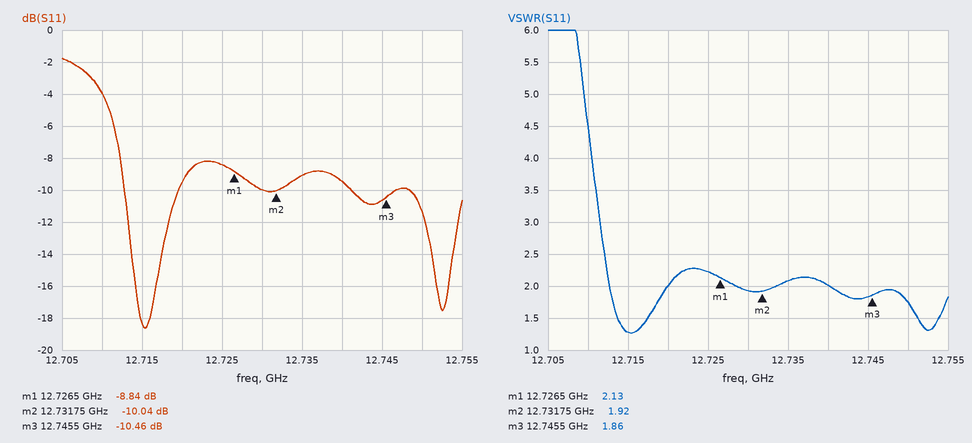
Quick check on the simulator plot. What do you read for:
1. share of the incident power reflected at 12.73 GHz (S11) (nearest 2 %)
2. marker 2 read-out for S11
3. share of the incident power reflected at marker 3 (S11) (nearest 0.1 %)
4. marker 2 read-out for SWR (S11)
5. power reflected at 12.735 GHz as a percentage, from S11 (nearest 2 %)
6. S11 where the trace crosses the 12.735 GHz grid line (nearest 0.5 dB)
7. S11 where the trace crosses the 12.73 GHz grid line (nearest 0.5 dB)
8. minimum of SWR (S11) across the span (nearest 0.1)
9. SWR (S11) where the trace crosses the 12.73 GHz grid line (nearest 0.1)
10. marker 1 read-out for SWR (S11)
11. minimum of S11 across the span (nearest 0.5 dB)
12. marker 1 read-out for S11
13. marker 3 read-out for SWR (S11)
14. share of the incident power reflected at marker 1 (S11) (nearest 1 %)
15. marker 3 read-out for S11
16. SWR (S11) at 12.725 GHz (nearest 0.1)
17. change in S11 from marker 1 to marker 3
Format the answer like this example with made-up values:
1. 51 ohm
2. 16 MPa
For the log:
1. 10 %
2. -10.04 dB
3. 9.0 %
4. 1.92
5. 12 %
6. -9.0 dB
7. -10.0 dB
8. 1.3
9. 1.9
10. 2.13
11. -18.5 dB
12. -8.84 dB
13. 1.86
14. 13 %
15. -10.46 dB
16. 2.2
17. -1.62 dB
